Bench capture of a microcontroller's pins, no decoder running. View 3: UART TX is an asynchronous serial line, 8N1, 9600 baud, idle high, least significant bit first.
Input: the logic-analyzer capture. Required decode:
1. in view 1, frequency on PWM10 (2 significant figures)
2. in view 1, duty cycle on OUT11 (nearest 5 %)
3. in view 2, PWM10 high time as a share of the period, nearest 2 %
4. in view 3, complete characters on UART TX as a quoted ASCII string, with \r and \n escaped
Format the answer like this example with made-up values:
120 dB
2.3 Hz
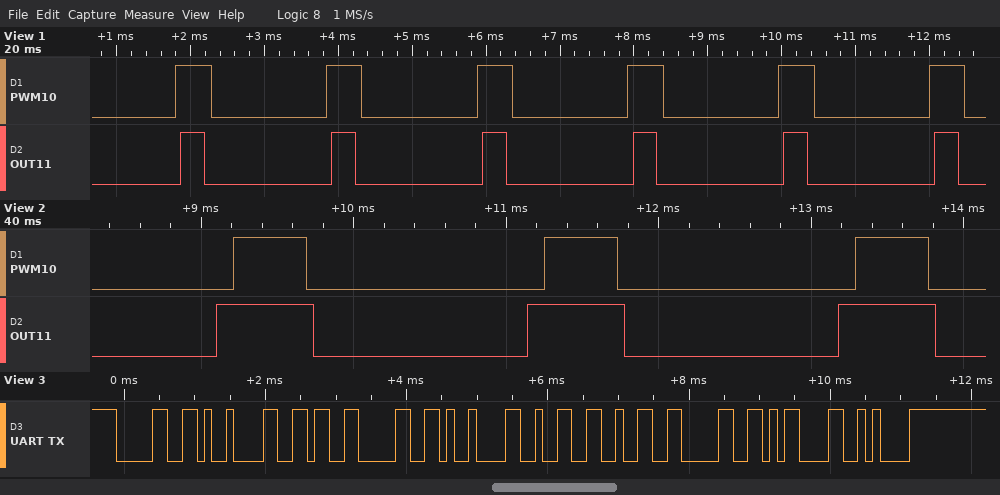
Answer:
490 Hz
15 %
24 %
"0\t60\t220\r\n"
